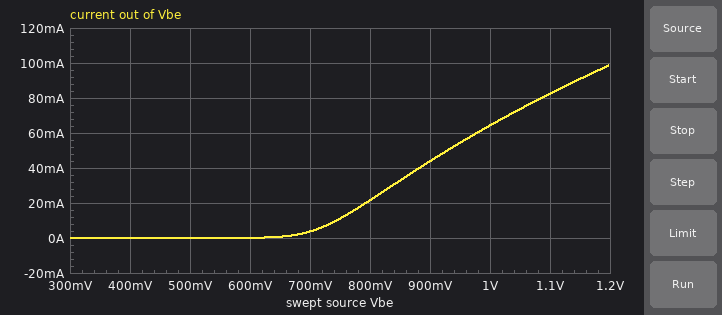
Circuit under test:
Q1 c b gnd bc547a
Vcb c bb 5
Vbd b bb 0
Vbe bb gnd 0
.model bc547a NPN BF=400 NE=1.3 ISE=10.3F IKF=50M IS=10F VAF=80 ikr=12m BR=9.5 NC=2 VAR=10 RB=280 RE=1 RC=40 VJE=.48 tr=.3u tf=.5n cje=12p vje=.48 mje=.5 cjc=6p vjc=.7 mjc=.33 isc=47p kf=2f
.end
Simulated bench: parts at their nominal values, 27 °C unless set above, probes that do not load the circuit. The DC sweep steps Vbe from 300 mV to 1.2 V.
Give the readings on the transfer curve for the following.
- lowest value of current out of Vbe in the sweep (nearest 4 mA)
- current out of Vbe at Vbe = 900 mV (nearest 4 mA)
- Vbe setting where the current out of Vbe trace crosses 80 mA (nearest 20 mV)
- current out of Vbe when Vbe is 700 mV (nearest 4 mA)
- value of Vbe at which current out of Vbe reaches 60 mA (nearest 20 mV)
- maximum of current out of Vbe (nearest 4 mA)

0 A
44 mA
1.08 V
4 mA
980 mV
100 mA
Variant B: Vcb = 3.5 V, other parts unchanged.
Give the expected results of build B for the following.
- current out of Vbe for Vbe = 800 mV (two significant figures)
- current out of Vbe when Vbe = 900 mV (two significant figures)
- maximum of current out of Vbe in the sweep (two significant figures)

21 mA
43 mA
97 mA
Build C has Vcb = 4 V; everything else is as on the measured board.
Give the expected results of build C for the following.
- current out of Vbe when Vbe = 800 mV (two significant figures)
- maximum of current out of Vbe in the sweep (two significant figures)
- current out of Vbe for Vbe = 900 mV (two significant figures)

21 mA
98 mA
43 mA
